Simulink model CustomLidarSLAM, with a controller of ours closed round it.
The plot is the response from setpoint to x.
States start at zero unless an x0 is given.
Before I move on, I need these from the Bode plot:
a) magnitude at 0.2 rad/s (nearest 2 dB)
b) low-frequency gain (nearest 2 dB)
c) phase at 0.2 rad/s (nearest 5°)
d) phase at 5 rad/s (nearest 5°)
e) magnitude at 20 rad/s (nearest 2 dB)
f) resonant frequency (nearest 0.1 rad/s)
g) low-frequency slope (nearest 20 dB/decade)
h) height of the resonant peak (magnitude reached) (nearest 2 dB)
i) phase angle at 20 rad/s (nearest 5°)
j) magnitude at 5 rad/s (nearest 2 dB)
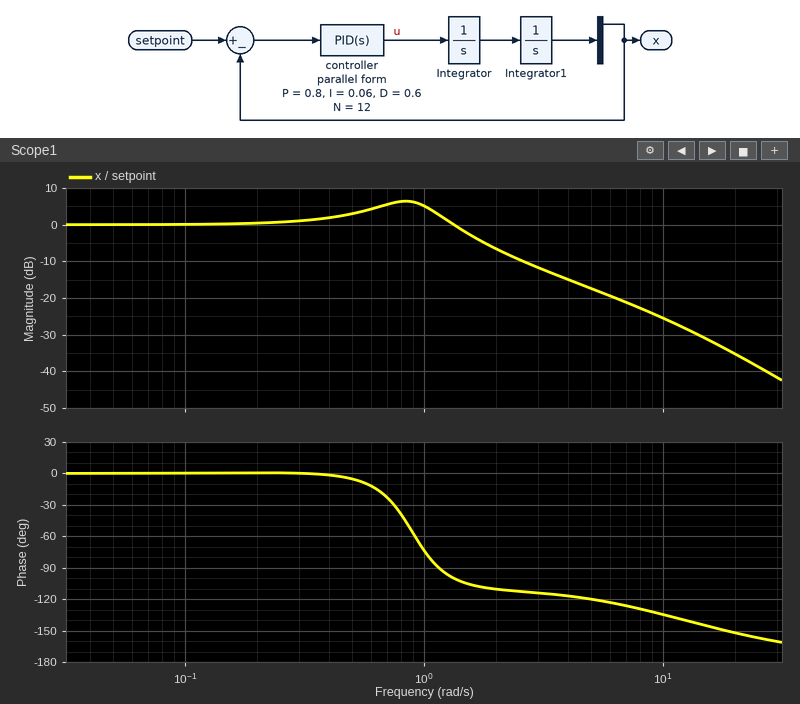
0 dB
0 dB
0°
-120°
-36 dB
0.8 rad/s
0 dB/decade
6 dB
-150°
-18 dB
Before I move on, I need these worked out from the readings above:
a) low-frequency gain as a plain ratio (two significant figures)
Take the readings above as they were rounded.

1.0
